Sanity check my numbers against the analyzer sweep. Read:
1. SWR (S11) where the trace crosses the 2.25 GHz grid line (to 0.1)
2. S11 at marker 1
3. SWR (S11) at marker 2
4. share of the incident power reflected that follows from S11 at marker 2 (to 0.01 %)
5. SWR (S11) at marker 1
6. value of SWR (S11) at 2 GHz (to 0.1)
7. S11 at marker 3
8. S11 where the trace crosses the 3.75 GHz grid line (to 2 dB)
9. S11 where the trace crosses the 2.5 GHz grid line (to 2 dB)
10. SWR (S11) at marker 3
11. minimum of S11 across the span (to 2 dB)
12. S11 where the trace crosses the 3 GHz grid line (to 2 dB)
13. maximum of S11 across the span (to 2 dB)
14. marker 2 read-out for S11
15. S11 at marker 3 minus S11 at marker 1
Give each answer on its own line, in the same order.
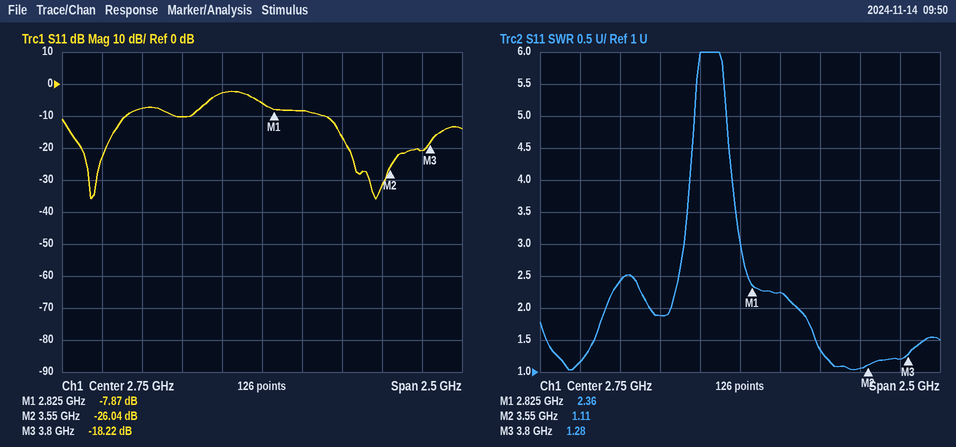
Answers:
1.9
-7.87 dB
1.11
0.25 %
2.36
2.4
-18.22 dB
-20 dB
-2 dB
1.28
-36 dB
-8 dB
-2 dB
-26.04 dB
-10.35 dB
